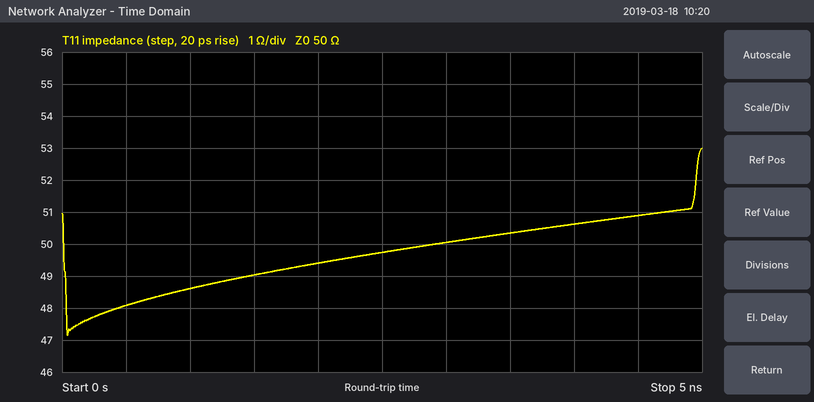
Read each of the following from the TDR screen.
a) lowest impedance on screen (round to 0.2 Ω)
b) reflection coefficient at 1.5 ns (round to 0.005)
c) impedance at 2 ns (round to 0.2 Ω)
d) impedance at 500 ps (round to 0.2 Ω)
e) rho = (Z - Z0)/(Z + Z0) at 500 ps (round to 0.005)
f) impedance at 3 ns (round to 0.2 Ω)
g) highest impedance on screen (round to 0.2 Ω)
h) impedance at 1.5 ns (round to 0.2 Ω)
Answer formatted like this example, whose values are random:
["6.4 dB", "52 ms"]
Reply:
["47.2 Ω", "-0.010", "49.4 Ω", "48.0 Ω", "-0.020", "50.0 Ω", "53.0 Ω", "49.0 Ω"]
